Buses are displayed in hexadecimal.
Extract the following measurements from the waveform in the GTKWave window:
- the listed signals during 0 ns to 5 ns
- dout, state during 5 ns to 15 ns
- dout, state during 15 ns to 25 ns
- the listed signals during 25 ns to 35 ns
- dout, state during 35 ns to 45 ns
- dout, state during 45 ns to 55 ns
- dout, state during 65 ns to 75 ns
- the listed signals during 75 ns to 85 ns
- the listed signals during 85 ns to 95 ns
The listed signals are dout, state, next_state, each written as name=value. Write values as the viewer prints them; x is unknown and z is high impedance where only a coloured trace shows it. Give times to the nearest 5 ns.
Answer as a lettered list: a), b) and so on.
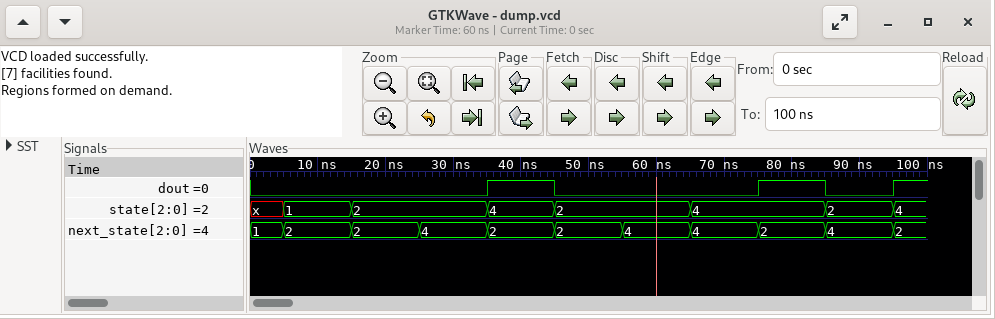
a) dout=0, state=x, next_state=1
b) dout=0, state=1
c) dout=0, state=2
d) dout=0, state=2, next_state=4
e) dout=1, state=4
f) dout=0, state=2
g) dout=0, state=4
h) dout=1, state=4, next_state=2
i) dout=0, state=2, next_state=4
